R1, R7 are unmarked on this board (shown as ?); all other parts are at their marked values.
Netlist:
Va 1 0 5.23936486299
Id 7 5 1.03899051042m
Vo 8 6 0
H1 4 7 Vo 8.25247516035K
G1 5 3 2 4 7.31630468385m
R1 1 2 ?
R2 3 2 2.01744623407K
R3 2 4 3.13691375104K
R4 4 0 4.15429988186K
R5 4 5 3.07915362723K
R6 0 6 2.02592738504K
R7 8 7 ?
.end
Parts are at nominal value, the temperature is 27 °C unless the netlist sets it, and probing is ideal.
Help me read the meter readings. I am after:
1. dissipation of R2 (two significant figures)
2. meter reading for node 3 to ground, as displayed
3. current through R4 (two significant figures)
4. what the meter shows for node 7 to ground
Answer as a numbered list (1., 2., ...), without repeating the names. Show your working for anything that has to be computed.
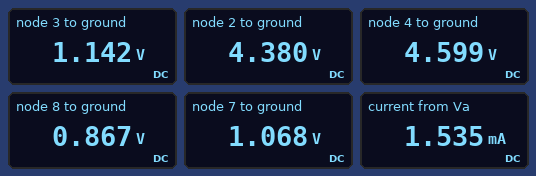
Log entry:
1. (4.38 V - 1.142 V)^2 / 2.017 kΩ = 5.2 mW
2. 1.142 V
3. (4.599 V) / 4.154 kΩ = 1.1 mA
4. 1.068 V
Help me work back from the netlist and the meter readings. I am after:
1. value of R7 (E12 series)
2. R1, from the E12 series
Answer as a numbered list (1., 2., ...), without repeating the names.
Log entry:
1. 470 Ω
2. 560 Ω
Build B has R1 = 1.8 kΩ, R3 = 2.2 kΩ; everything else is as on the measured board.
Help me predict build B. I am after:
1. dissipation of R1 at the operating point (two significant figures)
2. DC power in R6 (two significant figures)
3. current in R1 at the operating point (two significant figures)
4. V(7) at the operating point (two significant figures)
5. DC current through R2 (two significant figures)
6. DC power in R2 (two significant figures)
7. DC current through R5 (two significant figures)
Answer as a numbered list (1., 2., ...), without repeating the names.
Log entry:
1. 2.3 mW
2. 200 µW
3. 1.1 mA
4. 780 mV
5. 1.2 mA
6. 2.9 mW
7. 2.2 mA
